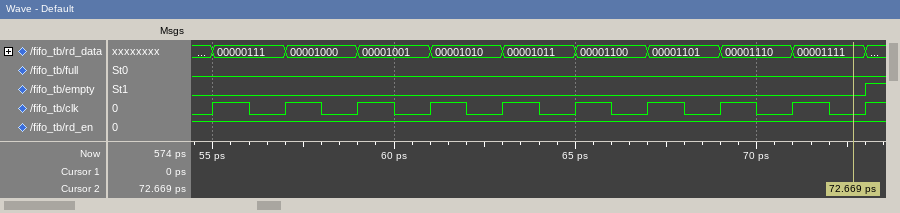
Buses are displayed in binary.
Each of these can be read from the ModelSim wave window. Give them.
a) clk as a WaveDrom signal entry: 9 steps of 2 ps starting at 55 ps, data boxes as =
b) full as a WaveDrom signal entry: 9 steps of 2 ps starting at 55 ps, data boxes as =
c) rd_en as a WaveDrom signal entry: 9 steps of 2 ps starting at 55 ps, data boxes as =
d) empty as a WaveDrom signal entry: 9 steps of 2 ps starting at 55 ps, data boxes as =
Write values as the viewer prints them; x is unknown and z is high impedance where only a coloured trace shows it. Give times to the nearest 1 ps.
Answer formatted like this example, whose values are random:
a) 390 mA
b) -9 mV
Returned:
a) {name: 'clk', wave: 'p........'}
b) {name: 'full', wave: '0........'}
c) {name: 'rd_en', wave: '1........'}
d) {name: 'empty', wave: '0........'}
